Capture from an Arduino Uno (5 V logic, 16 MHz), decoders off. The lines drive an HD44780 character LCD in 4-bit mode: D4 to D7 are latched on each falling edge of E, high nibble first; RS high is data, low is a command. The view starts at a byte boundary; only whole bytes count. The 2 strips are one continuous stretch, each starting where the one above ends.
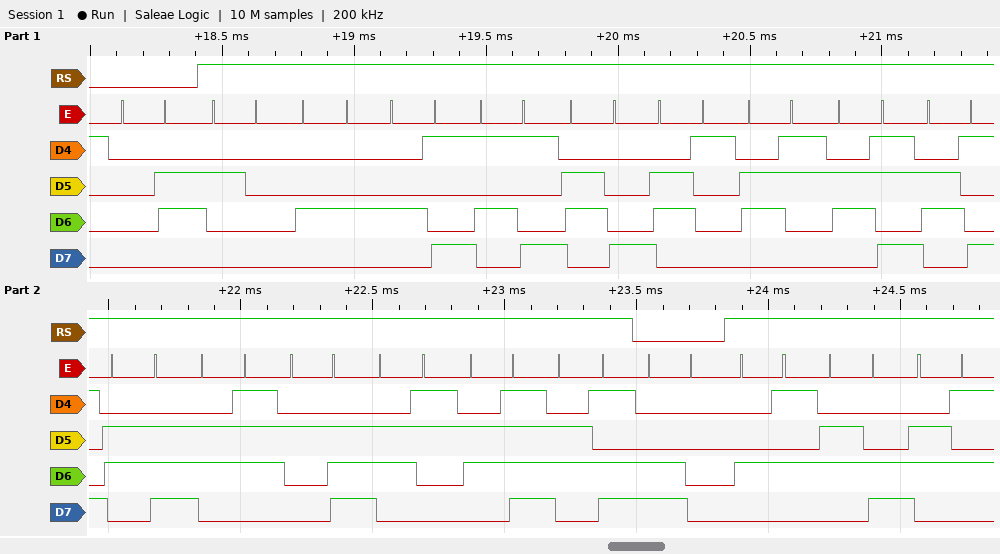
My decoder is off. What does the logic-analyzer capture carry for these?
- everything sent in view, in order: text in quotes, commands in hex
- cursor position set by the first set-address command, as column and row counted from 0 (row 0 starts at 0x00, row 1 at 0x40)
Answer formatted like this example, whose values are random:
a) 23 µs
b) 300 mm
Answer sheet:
a) 0x06 " DIYhacking.com" 0xC0 "Ele"
b) column 0, row 1
